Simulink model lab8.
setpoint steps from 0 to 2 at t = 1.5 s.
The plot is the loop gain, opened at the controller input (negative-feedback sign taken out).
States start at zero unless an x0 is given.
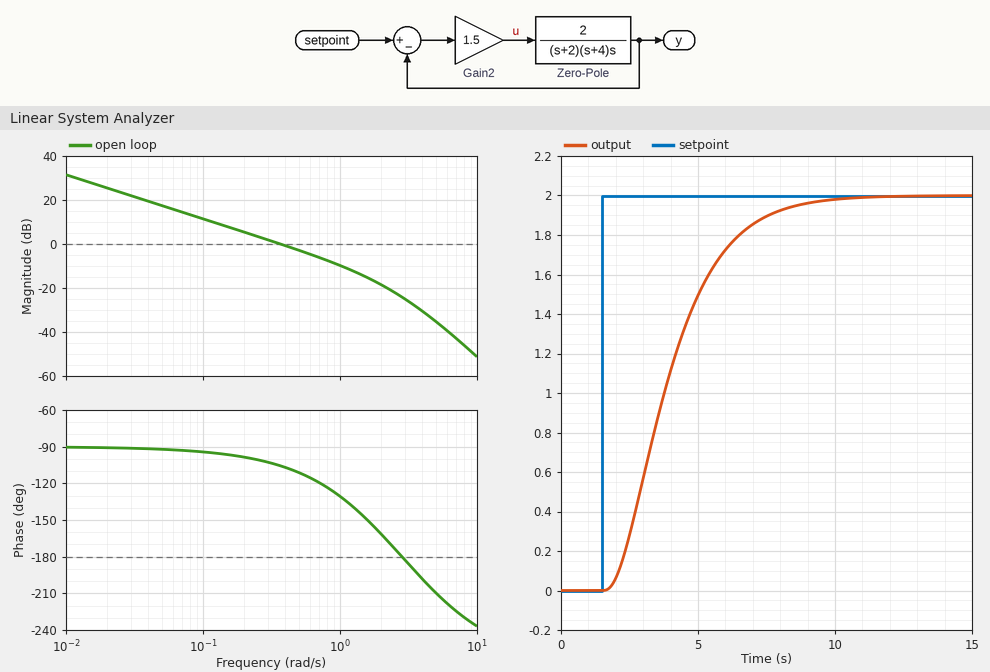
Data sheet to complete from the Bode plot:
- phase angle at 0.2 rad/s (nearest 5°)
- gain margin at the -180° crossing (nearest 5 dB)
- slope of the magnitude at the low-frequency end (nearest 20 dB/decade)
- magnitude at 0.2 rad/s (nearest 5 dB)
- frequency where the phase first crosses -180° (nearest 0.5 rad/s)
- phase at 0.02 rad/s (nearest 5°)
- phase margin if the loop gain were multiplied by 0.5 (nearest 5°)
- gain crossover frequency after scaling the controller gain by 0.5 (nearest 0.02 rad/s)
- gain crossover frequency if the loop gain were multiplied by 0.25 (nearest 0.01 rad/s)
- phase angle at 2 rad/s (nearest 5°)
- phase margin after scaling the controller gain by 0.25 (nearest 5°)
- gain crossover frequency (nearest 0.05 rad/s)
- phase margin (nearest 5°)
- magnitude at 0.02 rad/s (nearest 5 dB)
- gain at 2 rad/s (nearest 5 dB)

-100°
25 dB
-20 dB/decade
5 dB
3.0 rad/s
-90°
80°
0.18 rad/s
0.09 rad/s
-160°
85°
0.35 rad/s
75°
25 dB
-20 dB
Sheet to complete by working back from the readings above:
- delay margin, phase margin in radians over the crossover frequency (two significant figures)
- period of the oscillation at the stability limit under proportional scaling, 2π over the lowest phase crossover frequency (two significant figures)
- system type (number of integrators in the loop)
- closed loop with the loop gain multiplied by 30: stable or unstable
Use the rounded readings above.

3.7 s
2.1 s
1
unstable
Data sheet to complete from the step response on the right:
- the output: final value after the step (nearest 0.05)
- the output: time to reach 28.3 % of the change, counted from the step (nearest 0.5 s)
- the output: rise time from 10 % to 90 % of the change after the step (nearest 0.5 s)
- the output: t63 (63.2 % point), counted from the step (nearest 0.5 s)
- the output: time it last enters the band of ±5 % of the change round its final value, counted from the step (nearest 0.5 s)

2.00
1.5 s
4.0 s
3.0 s
6.0 s
